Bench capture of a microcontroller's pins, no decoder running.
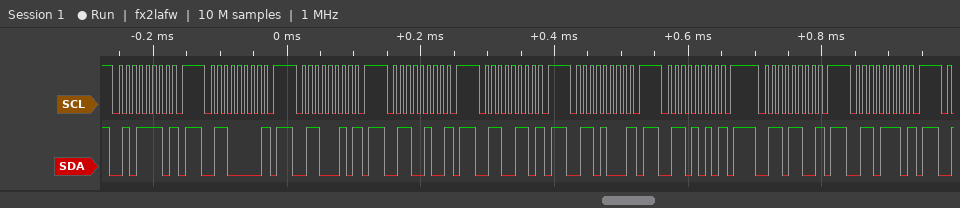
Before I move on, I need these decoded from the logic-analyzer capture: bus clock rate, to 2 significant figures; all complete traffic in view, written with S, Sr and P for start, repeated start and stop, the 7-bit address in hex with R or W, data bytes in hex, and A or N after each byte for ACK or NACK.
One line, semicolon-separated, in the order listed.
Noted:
100 kHz; S 2FW N P S 30W N P S 31W N P S 32W N P S 33W N P S 34W N P S 35W N P S 36W N P S 37W N P
